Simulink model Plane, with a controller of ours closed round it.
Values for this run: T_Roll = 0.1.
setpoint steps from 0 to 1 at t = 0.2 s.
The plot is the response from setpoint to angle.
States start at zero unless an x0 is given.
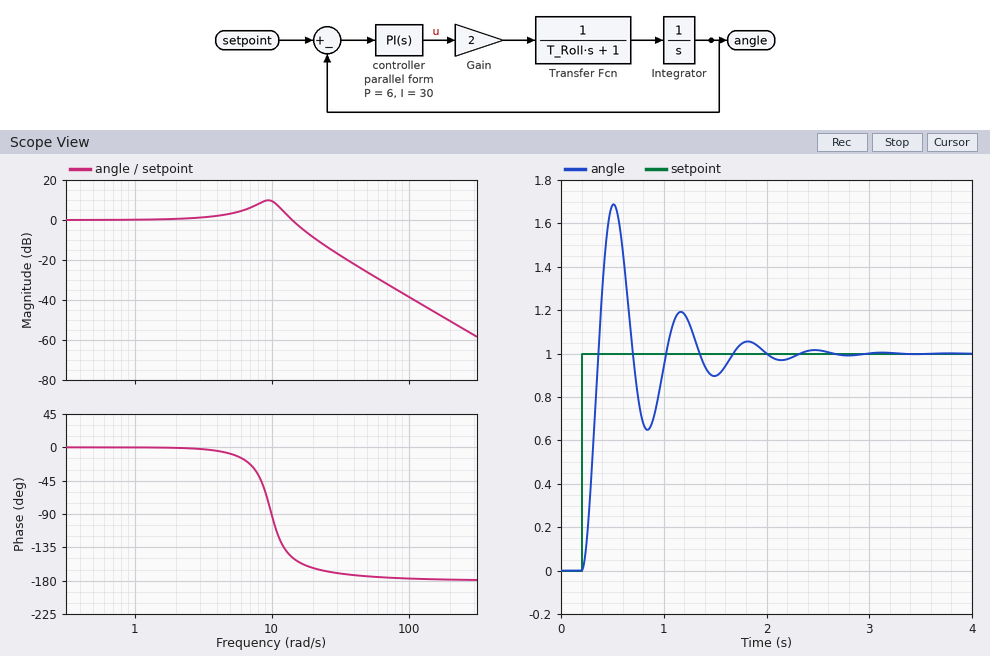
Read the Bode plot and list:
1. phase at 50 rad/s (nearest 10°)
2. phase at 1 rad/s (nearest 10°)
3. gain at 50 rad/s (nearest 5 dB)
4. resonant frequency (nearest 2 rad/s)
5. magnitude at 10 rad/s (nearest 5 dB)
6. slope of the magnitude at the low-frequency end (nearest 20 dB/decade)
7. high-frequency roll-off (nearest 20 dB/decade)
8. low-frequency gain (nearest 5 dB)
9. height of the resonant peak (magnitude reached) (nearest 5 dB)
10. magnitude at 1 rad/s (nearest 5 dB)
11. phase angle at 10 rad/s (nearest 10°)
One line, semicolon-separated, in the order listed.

-170°; 0°; -25 dB; 10 rad/s; 10 dB; 0 dB/decade; -40 dB/decade; 0 dB; 10 dB; 0 dB; -90°
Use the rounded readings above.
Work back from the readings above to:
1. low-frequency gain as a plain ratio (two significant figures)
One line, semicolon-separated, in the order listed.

1.0
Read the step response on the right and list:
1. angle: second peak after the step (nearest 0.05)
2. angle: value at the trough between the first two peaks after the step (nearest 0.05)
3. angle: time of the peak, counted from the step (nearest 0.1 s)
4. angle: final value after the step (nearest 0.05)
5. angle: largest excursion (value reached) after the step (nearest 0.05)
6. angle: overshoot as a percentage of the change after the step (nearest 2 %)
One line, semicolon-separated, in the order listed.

1.20; 0.65; 0.3 s; 1.00; 1.70; 68 %
